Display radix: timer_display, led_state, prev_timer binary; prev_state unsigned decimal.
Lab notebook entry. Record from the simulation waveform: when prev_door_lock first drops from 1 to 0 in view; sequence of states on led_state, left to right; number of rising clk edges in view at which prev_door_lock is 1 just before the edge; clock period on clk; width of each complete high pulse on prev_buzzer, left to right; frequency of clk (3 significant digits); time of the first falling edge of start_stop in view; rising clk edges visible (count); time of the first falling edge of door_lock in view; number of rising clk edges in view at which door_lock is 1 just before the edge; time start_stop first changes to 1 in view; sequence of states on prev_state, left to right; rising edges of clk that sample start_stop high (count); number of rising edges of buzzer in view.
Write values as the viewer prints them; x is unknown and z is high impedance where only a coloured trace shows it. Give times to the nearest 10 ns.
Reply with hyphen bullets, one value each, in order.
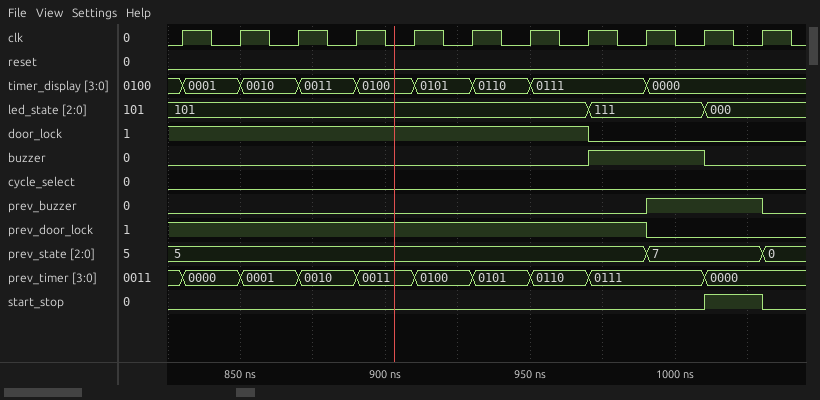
- 990 ns
- 101, 111, 000
- 9
- 20 ns
- 40 ns
- 50.0 MHz
- 1030 ns
- 11
- 970 ns
- 8
- 1010 ns
- 5, 7, 0
- 1
- 1
